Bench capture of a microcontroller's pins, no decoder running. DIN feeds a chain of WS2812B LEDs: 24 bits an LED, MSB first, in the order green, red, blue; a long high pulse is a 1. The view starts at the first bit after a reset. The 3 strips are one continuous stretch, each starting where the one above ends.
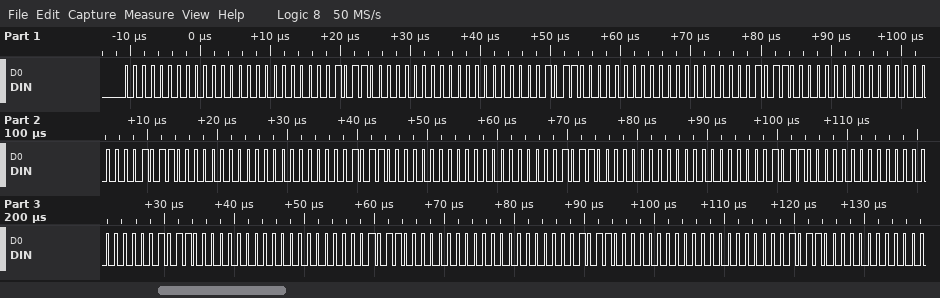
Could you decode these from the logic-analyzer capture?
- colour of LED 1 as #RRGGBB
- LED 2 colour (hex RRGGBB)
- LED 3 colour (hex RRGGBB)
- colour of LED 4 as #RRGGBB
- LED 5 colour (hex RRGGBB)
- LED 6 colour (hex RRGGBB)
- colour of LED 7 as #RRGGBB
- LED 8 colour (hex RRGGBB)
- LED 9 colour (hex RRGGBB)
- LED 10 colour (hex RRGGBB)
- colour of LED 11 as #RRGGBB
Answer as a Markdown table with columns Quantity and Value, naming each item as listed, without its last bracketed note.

| Quantity | Value |
|---|---|
| colour of LED 1 as #RRGGBB | #000000 |
| LED 2 colour | #00B000 |
| LED 3 colour | #00B000 |
| colour of LED 4 as #RRGGBB | #00B000 |
| LED 5 colour | #00B000 |
| LED 6 colour | #00B000 |
| colour of LED 7 as #RRGGBB | #00B000 |
| LED 8 colour | #00B000 |
| LED 9 colour | #00B000 |
| LED 10 colour | #00B000 |
| colour of LED 11 as #RRGGBB | #00B000 |
